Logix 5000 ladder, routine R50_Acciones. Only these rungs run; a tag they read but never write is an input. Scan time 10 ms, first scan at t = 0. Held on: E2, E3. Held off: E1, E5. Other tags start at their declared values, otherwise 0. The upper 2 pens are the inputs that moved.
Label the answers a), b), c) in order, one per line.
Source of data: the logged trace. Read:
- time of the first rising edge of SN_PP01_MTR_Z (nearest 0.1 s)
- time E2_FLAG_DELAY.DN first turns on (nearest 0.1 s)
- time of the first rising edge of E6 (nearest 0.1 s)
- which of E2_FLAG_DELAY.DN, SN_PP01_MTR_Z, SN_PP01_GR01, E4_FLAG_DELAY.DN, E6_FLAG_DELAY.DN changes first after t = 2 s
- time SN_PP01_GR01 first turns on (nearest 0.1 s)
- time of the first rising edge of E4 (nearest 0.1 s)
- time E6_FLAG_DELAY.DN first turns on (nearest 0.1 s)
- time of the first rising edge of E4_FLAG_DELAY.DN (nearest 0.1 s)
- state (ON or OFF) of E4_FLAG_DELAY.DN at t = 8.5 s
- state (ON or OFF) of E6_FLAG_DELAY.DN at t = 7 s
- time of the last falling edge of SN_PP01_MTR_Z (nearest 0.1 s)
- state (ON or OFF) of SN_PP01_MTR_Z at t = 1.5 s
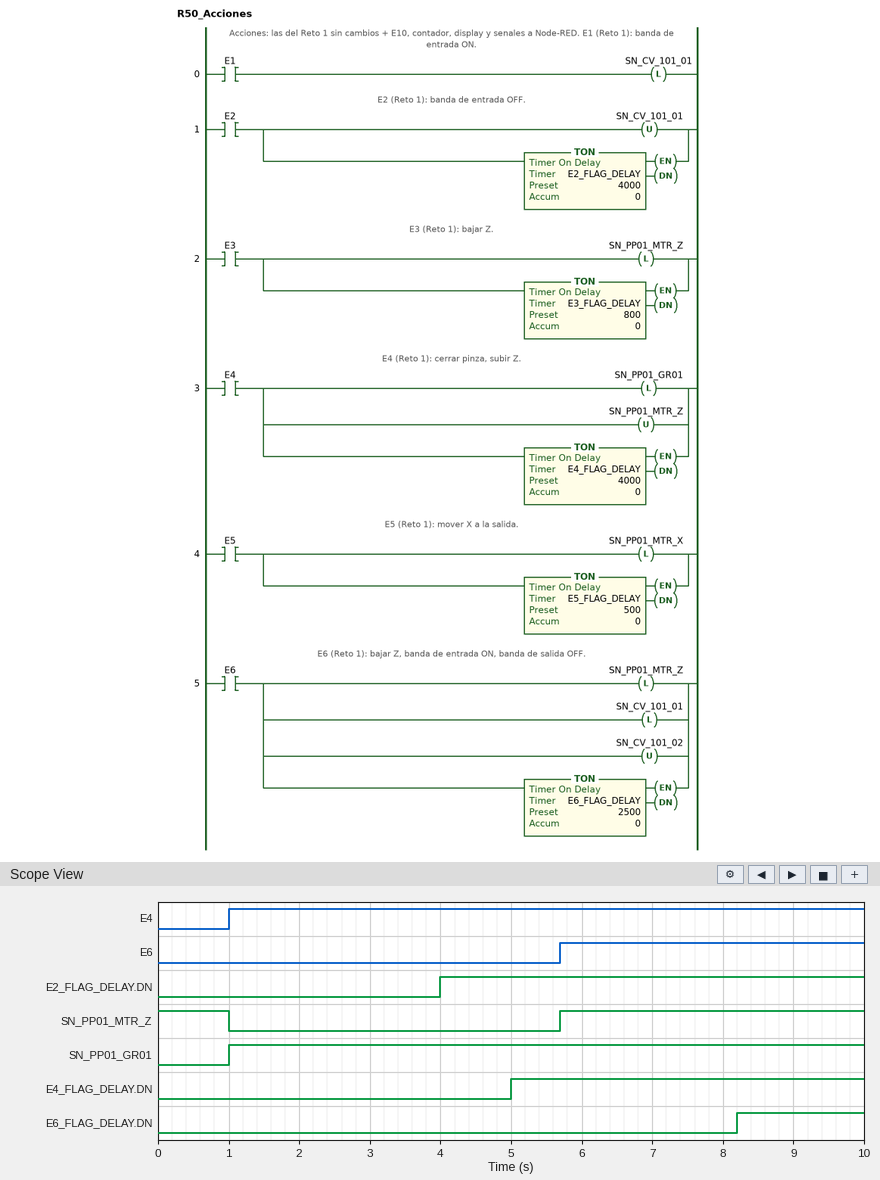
a) 5.7 s
b) 4.0 s
c) 5.7 s
d) E2_FLAG_DELAY.DN
e) 1.0 s
f) 1.0 s
g) 8.2 s
h) 5.0 s
i) ON
j) OFF
k) 1.0 s
l) OFF
